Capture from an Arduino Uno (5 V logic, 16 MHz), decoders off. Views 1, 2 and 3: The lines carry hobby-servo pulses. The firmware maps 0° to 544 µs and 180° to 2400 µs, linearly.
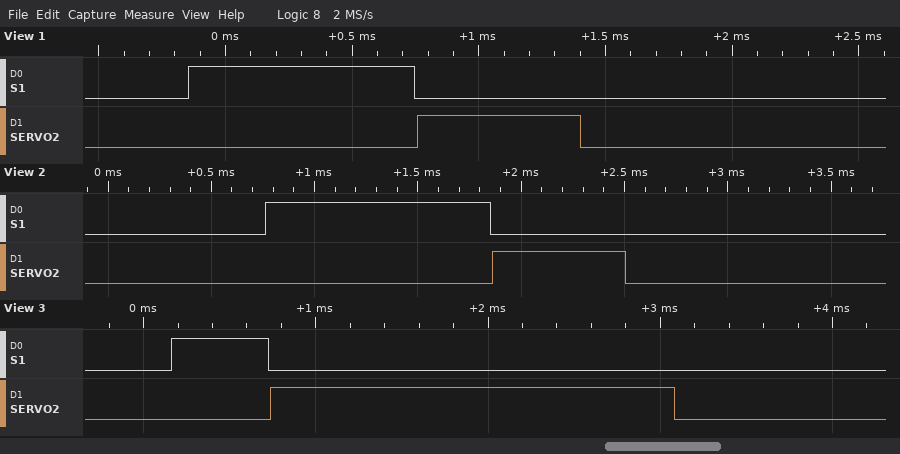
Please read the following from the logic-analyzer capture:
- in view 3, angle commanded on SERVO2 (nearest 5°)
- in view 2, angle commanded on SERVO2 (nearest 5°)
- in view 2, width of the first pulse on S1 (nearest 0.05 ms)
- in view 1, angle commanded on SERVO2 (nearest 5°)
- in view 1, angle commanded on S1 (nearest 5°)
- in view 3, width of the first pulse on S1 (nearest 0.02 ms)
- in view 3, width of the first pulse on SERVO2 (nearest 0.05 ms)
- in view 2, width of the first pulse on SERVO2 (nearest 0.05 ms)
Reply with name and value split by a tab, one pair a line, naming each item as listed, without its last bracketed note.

in view 3, angle commanded on SERVO2	175°
in view 2, angle commanded on SERVO2	10°
in view 2, width of the first pulse on S1	1.10 ms
in view 1, angle commanded on SERVO2	10°
in view 1, angle commanded on S1	35°
in view 3, width of the first pulse on S1	0.56 ms
in view 3, width of the first pulse on SERVO2	2.35 ms
in view 2, width of the first pulse on SERVO2	0.65 ms
